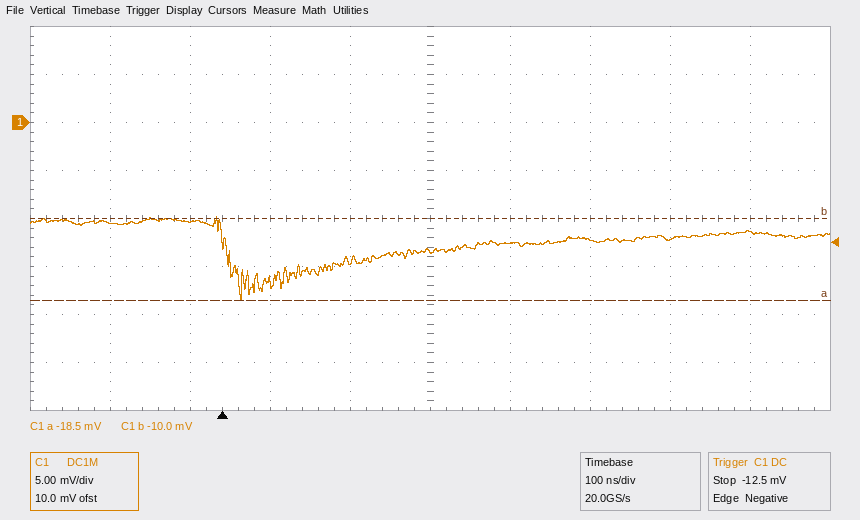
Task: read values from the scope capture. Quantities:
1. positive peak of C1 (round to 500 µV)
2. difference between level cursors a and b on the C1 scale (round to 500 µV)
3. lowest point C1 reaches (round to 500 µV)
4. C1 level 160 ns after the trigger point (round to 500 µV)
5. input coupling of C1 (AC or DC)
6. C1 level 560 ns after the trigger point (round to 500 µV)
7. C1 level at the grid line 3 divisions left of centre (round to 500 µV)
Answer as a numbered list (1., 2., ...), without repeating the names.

1. -10.0 mV
2. 8.5 mV
3. -18.5 mV
4. -14.5 mV
5. DC
6. -12.0 mV
7. -10.5 mV
